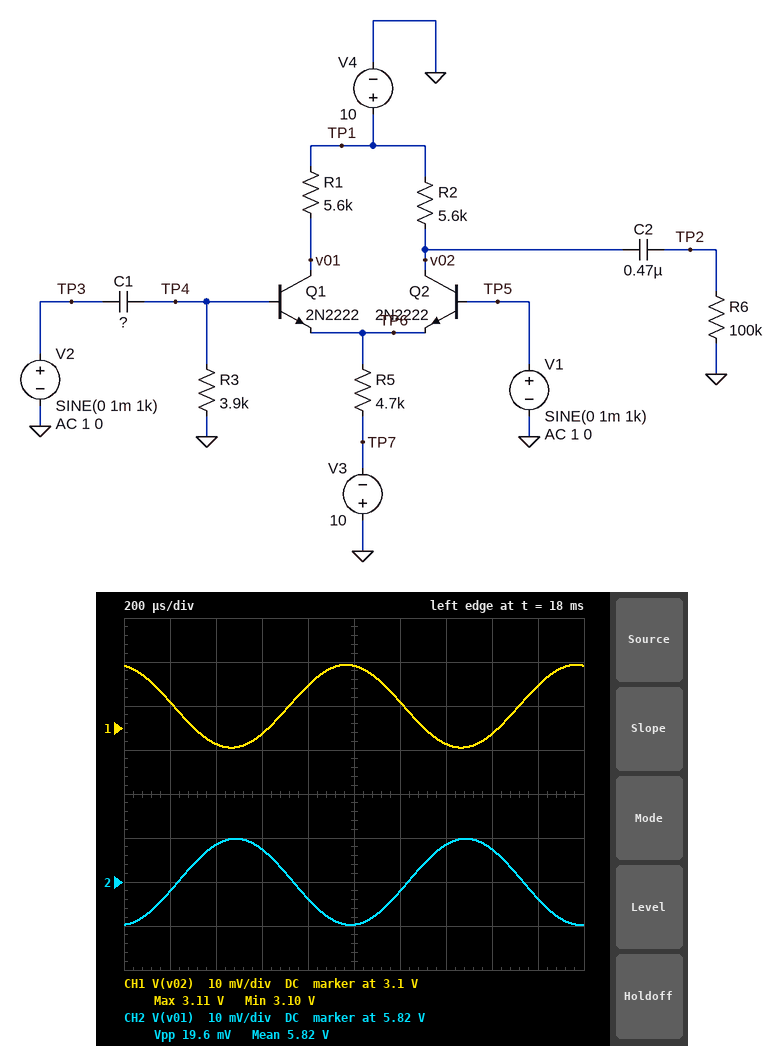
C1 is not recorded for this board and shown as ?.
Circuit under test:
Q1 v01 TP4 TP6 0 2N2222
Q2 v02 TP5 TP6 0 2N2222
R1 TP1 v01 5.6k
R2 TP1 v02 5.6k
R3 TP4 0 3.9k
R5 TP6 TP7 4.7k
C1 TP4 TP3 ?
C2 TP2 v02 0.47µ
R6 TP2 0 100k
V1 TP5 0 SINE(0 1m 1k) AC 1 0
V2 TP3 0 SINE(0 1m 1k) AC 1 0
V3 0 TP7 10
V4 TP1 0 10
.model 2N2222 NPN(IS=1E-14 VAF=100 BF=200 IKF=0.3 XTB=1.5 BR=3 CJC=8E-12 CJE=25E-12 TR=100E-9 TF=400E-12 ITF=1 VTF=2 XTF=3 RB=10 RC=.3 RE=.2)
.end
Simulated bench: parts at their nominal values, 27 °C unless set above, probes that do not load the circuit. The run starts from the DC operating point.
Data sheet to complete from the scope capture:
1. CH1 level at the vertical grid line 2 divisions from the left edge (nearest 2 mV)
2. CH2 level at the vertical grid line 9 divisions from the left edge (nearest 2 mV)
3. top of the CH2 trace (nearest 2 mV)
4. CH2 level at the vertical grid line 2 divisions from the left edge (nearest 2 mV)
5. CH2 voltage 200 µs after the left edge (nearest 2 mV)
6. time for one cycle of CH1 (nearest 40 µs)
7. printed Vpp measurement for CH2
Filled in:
3.096 V
5.816 V
5.830 V
5.828 V
5.818 V
1.00 ms
19.6 mV
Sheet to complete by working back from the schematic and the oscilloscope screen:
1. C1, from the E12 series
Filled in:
390 nF
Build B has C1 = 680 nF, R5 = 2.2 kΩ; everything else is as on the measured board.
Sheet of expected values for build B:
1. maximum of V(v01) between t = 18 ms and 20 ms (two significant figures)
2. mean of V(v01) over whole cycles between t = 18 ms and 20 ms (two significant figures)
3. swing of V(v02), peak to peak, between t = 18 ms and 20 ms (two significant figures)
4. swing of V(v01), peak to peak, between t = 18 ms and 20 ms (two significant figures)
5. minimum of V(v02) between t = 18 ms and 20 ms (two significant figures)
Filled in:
710 mV
700 mV
2.0 mV
14 mV
-680 mV
